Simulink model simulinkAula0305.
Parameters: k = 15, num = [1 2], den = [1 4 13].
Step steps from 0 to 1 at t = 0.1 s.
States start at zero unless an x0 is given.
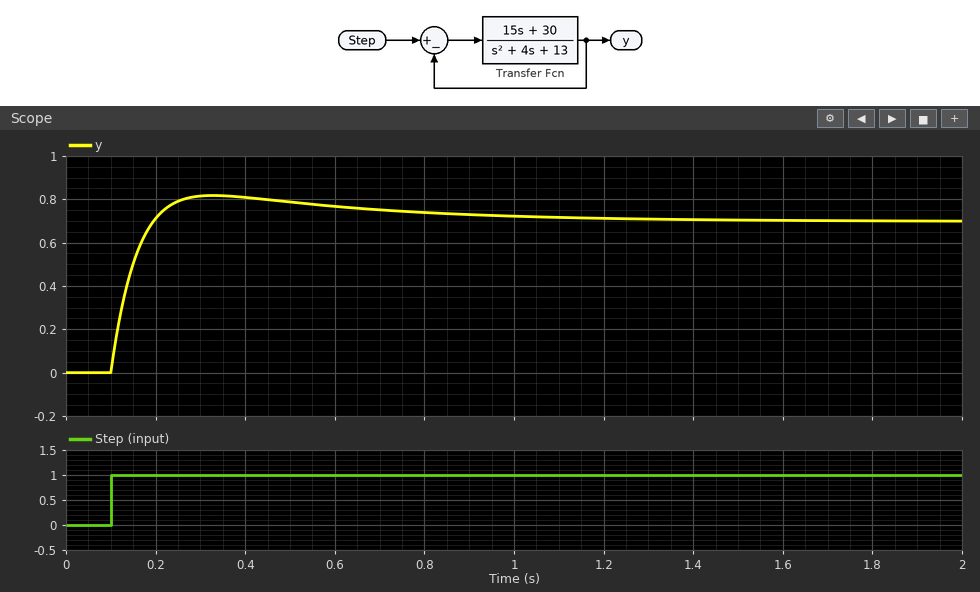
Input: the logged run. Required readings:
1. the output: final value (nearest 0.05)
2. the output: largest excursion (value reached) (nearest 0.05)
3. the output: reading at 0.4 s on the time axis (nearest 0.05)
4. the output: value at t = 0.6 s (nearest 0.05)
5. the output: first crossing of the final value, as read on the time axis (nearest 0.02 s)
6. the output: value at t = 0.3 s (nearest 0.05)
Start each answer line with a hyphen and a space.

- 0.70
- 0.80
- 0.80
- 0.75
- 0.20 s
- 0.80
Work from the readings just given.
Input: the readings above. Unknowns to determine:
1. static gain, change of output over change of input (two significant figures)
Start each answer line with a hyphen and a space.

- 0.70
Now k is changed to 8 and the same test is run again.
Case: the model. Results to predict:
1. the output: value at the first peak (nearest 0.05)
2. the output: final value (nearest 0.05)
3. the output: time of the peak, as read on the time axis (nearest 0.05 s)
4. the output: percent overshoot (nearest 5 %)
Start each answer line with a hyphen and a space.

- 0.70
- 0.55
- 0.40 s
- 25 %
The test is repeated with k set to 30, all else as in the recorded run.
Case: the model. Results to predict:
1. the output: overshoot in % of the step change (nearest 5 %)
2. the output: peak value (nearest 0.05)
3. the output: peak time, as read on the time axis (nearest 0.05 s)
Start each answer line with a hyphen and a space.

- 10 %
- 0.90
- 0.25 s
